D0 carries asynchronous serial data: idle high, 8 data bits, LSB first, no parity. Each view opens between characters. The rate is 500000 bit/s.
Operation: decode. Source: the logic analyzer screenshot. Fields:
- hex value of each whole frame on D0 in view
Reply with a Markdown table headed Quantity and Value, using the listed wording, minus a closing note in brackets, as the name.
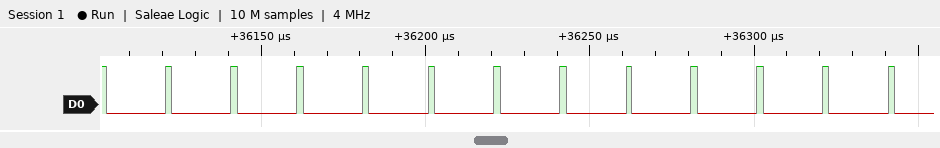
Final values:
| Quantity | Value |
|---|---|
| hex value of each whole frame on D0 in view | 00, 00, 00, 00, 00, 00, 00, 00, 00, 00, 00, 00 |
